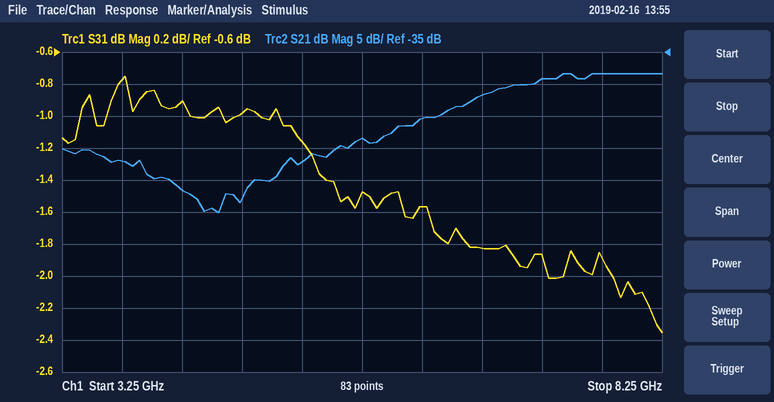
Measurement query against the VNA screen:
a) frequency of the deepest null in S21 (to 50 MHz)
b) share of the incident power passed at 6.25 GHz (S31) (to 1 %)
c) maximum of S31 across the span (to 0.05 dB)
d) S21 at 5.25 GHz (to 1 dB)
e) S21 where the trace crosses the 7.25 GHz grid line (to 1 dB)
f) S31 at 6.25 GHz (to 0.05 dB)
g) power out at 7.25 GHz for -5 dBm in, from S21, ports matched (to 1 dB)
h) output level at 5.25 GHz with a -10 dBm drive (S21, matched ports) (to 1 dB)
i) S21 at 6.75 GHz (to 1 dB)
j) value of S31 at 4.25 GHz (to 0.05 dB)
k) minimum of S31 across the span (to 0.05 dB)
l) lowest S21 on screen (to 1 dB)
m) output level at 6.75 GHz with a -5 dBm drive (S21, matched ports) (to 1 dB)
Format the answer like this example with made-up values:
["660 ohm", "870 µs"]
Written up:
["4.55 GHz", "70 %", "-0.75 dB", "-52 dB", "-39 dB", "-1.55 dB", "-44 dBm", "-62 dBm", "-42 dB", "-0.90 dB", "-2.35 dB", "-60 dB", "-47 dBm"]
